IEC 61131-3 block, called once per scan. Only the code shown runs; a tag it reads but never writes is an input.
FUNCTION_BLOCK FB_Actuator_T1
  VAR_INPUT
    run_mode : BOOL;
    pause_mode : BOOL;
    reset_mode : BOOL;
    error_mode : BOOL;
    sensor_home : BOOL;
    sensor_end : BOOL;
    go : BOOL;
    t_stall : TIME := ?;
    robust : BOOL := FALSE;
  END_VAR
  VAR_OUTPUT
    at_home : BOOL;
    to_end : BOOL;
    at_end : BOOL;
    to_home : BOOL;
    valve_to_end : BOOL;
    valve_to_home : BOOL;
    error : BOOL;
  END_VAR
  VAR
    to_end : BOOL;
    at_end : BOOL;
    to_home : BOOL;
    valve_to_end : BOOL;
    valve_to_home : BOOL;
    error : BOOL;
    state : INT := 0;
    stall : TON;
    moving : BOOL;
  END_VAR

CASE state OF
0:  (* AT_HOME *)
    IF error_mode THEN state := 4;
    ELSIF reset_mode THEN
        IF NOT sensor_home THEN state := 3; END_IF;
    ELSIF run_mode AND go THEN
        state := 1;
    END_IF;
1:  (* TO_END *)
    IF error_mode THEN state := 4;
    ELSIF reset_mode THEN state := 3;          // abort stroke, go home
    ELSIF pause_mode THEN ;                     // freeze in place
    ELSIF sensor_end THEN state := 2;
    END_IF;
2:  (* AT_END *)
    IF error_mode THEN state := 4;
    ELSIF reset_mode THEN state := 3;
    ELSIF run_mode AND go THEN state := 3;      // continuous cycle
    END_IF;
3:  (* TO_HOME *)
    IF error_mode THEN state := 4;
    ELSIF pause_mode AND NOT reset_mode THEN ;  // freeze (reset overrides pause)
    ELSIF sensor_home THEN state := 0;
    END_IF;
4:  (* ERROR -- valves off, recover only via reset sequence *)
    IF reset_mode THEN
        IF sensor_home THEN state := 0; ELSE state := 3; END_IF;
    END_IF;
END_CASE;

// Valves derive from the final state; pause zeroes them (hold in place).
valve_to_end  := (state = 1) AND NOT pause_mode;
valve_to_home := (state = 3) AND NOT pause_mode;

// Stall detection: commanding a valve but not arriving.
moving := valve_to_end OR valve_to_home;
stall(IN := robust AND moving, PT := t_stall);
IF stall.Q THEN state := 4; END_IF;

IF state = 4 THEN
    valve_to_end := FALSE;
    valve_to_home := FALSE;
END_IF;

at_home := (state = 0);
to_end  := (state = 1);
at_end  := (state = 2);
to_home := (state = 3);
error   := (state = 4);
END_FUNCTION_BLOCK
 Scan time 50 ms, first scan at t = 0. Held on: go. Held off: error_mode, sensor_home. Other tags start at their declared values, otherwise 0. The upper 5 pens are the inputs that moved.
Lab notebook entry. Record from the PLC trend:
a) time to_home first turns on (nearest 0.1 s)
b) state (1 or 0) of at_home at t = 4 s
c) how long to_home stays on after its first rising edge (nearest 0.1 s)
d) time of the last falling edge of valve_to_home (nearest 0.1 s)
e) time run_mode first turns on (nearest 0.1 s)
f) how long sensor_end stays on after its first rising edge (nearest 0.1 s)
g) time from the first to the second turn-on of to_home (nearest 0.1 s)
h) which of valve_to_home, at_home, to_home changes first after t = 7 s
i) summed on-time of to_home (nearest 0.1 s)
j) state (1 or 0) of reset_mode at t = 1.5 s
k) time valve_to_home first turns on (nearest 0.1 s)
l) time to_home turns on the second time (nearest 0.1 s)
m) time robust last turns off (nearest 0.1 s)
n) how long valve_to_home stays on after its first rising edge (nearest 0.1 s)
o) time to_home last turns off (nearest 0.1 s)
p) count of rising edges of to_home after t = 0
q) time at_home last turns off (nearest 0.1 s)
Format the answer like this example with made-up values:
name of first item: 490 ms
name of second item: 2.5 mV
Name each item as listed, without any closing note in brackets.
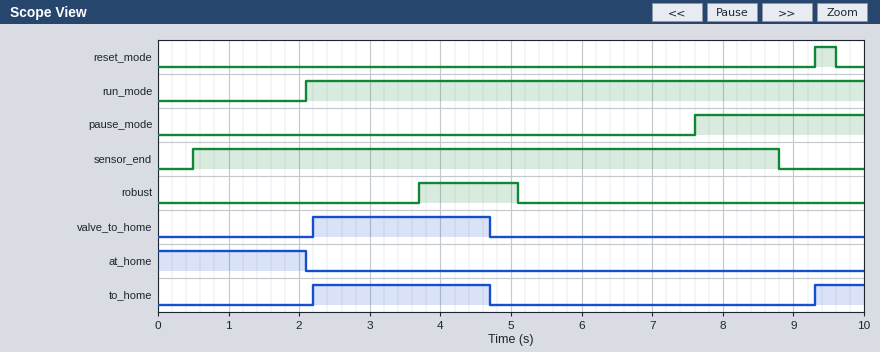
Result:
time to_home first turns on: 2.2 s
state (1 or 0) of at_home at t = 4 s: 0
how long to_home stays on after its first rising edge: 2.5 s
time of the last falling edge of valve_to_home: 4.7 s
time run_mode first turns on: 2.1 s
how long sensor_end stays on after its first rising edge: 8.3 s
time from the first to the second turn-on of to_home: 7.1 s
which of valve_to_home, at_home, to_home changes first after t = 7 s: to_home
summed on-time of to_home: 3.2 s
state (1 or 0) of reset_mode at t = 1.5 s: 0
time valve_to_home first turns on: 2.2 s
time to_home turns on the second time: 9.3 s
time robust last turns off: 5.1 s
how long valve_to_home stays on after its first rising edge: 2.5 s
time to_home last turns off: 4.7 s
count of rising edges of to_home after t = 0: 2
time at_home last turns off: 2.1 s
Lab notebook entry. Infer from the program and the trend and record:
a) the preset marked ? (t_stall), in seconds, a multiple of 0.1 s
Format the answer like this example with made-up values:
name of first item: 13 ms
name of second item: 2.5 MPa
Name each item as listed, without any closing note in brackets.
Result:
the preset marked ? (t_stall), in seconds, a multiple of 0.1 s: 1.0 s
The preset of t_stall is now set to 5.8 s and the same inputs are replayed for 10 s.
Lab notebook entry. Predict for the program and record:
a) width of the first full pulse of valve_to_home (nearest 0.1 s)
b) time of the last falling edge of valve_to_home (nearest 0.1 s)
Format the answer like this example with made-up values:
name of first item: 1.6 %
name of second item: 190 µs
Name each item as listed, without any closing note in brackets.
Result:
width of the first full pulse of valve_to_home: 5.4 s
time of the last falling edge of valve_to_home: 7.6 s
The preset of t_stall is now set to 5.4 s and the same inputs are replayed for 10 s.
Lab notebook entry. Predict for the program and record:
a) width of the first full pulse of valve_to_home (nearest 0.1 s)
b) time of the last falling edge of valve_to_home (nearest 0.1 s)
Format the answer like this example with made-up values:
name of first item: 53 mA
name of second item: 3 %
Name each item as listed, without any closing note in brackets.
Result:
width of the first full pulse of valve_to_home: 5.4 s
time of the last falling edge of valve_to_home: 7.6 s
